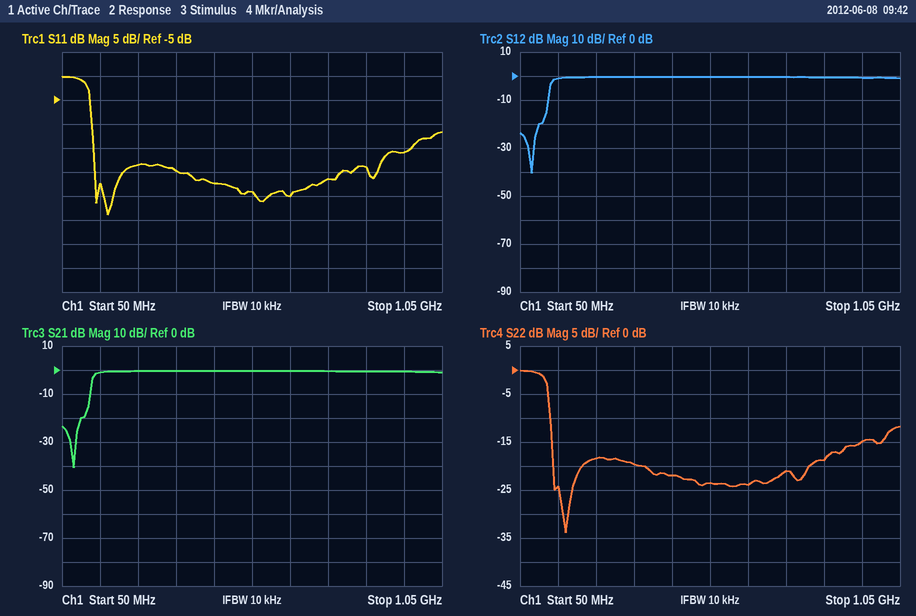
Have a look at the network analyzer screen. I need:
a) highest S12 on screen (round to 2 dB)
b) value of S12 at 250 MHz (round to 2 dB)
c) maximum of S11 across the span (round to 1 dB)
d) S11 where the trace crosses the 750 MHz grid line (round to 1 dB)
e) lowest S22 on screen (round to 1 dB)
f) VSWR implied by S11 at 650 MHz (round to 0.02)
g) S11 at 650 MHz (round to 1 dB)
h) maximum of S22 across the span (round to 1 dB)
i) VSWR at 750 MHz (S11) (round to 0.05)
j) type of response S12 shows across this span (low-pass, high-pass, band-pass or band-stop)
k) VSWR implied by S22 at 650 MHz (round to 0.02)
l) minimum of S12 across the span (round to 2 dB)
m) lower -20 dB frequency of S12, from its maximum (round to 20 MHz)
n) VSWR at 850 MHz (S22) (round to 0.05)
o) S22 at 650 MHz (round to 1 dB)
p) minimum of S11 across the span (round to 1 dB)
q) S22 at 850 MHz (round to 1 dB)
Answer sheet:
0 dB
0 dB
0 dB
-21 dB
-34 dB
1.12
-25 dB
0 dB
1.20
high-pass
1.14
-40 dB
100 MHz
1.25
-24 dB
-29 dB
-19 dB
